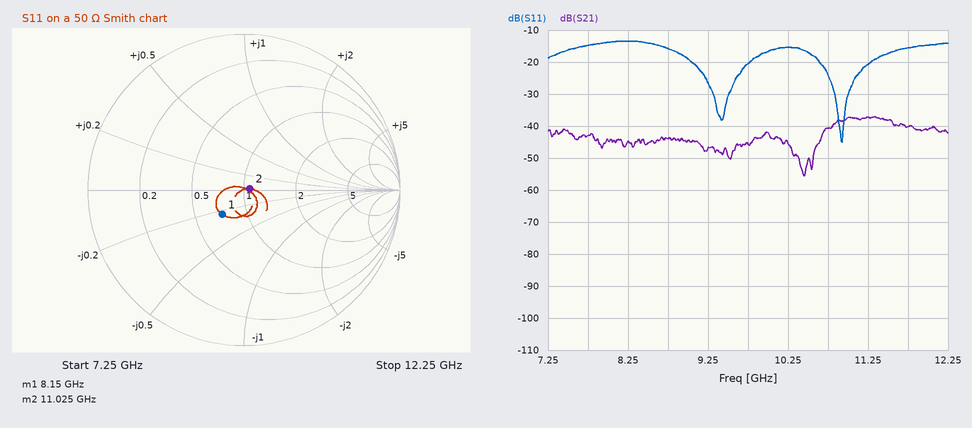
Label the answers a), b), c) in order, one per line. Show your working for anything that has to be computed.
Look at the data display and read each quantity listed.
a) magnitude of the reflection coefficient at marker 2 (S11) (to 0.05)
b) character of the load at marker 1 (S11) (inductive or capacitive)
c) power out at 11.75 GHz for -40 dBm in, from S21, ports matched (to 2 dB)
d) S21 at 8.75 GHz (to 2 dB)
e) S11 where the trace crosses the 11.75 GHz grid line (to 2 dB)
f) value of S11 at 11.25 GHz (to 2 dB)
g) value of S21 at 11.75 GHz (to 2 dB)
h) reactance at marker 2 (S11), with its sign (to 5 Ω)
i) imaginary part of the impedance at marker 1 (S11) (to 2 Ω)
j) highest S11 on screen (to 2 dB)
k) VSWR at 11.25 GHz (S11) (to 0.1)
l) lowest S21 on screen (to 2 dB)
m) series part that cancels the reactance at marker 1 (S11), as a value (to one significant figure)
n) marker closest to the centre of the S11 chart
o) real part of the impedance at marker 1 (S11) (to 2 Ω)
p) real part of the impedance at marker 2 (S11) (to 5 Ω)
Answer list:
a) 0.05
b) capacitive
c) -40 dBm + (-40 dB) = -80 dBm
d) -44 dB
e) -16 dB
f) -20 dB
g) -40 dB
h) 0 Ω
i) -12 Ω
j) -14 dB
k) |Γ| = 10^(-20/20) = 0.1000; VSWR = (1 + 0.1000)/(1 − 0.1000) ≈ 1.2
l) -56 dB
m) L = 12 Ω/(2π × 8.15 GHz) ≈ 234 pH, so 200 pH to one significant figure
n) marker 2
o) 36 Ω
p) 55 Ω
